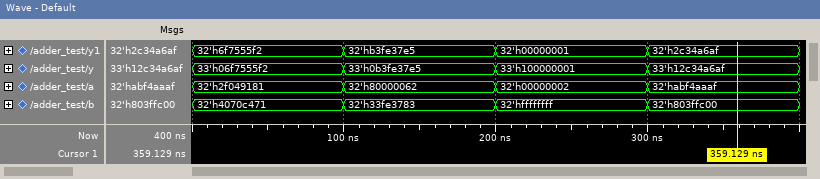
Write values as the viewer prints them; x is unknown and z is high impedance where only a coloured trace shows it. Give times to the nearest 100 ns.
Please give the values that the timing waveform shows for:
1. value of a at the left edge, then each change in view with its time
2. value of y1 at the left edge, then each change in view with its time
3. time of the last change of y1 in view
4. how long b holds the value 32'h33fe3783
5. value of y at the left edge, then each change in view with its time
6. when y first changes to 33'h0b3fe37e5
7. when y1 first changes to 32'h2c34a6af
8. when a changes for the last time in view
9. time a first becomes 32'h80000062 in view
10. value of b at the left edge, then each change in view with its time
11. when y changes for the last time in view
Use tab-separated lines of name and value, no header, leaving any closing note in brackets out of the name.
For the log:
value of a at the left edge, then each change in view with its time	32'h2f049181, 32'h80000062 at 100 ns, 32'h00000002 at 200 ns, 32'habf4aaaf at 300 ns
value of y1 at the left edge, then each change in view with its time	32'h6f7555f2, 32'hb3fe37e5 at 100 ns, 32'h00000001 at 200 ns, 32'h2c34a6af at 300 ns
time of the last change of y1 in view	300 ns
how long b holds the value 32'h33fe3783	100 ns
value of y at the left edge, then each change in view with its time	33'h06f7555f2, 33'h0b3fe37e5 at 100 ns, 33'h100000001 at 200 ns, 33'h12c34a6af at 300 ns
when y first changes to 33'h0b3fe37e5	100 ns
when y1 first changes to 32'h2c34a6af	300 ns
when a changes for the last time in view	300 ns
time a first becomes 32'h80000062 in view	100 ns
value of b at the left edge, then each change in view with its time	32'h4070c471, 32'h33fe3783 at 100 ns, 32'hffffffff at 200 ns, 32'h803ffc00 at 300 ns
when y changes for the last time in view	300 ns
